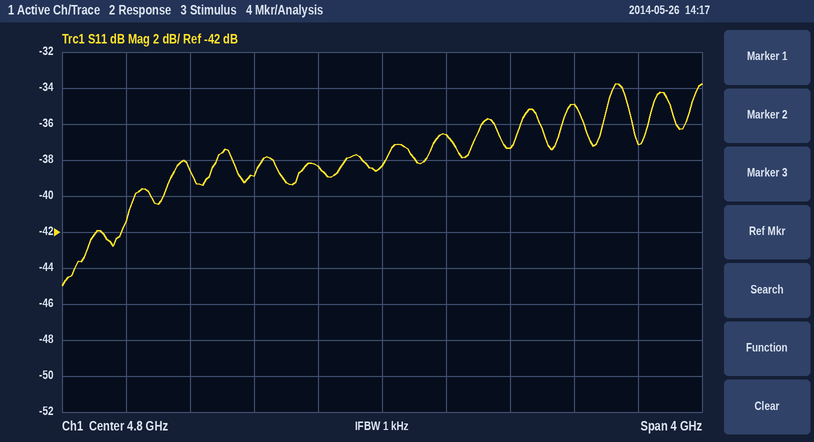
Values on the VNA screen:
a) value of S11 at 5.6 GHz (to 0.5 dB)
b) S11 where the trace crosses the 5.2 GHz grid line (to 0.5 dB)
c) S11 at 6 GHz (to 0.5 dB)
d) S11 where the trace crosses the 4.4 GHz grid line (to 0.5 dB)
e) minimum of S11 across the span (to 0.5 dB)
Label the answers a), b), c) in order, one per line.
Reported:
a) -37.5 dB
b) -36.5 dB
c) -35.0 dB
d) -38.5 dB
e) -45.0 dB
